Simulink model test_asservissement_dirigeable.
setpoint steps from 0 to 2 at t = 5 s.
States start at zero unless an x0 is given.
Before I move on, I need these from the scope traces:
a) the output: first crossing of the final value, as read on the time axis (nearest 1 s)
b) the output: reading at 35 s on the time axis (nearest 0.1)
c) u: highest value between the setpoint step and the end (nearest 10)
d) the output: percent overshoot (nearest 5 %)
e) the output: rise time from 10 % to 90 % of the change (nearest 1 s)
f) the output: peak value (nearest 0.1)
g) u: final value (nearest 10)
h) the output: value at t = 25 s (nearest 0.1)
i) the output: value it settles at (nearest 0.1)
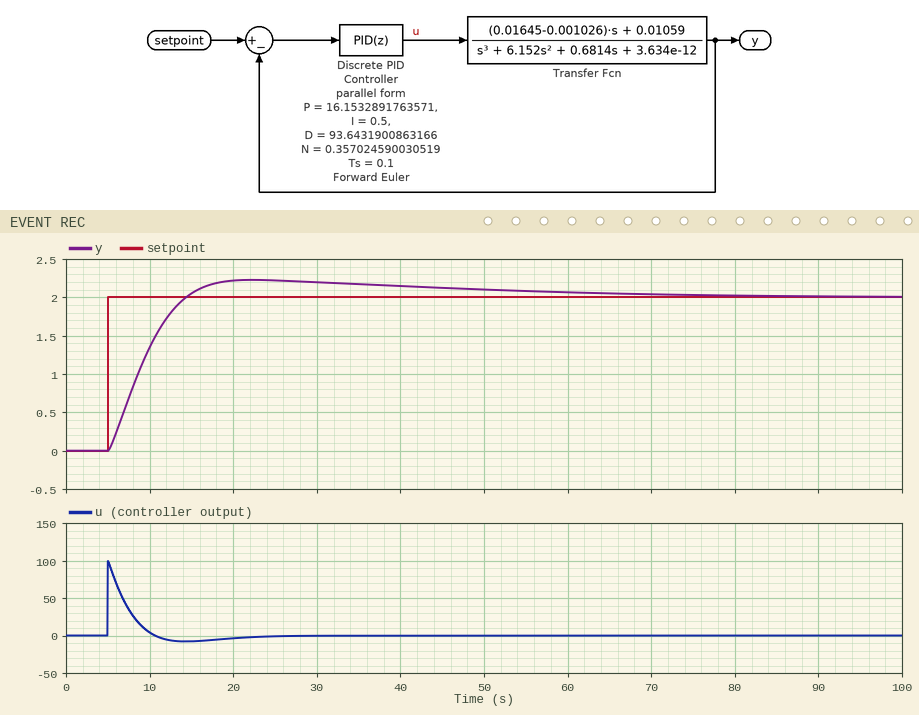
14 s
2.2
100
10 %
7 s
2.2
0
2.2
2.0
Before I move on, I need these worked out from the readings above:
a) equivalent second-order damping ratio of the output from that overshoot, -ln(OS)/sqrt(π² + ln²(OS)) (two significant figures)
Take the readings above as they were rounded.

0.59
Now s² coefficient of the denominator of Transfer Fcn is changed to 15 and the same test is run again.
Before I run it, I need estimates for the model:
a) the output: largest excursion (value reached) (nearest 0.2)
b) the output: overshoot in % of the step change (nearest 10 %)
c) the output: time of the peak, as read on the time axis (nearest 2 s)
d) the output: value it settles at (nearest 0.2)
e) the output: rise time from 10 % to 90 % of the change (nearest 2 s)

2.6
30 %
30 s
2.0
10 s
